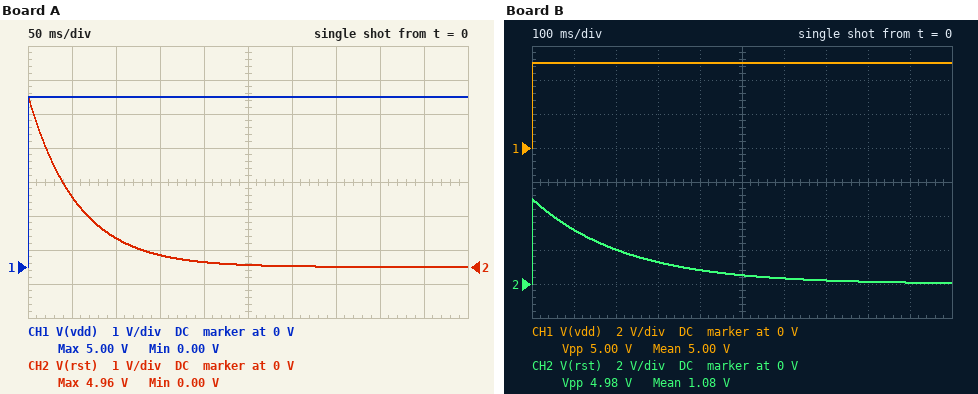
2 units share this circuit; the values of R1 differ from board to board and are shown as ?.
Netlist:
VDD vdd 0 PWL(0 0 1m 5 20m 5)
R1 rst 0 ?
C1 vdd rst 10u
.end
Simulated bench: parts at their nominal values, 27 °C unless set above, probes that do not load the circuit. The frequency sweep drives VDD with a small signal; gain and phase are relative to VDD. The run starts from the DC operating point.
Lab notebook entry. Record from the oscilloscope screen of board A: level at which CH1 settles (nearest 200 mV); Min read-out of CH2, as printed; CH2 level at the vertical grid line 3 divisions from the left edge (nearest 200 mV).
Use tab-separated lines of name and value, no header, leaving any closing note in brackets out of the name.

level at which CH1 settles	5.0 V
Min read-out of CH2, as printed	0.00 V
CH2 level at the vertical grid line 3 divisions from the left edge	400 mV
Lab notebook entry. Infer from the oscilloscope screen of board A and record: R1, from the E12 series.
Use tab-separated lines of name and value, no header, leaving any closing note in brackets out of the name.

R1, from the E12 series	5.6 kΩ
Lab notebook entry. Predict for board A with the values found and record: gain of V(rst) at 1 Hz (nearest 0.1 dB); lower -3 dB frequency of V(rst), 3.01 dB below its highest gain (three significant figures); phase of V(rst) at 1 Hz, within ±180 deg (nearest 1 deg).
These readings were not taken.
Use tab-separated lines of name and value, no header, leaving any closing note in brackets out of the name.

gain of V(rst) at 1 Hz	-9.6 dB
lower -3 dB frequency of V(rst), 3.01 dB below its highest gain	2.84 Hz
phase of V(rst) at 1 Hz, within ±180 deg	71 deg
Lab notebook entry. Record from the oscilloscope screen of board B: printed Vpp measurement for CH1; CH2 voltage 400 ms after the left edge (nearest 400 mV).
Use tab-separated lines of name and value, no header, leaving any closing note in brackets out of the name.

printed Vpp measurement for CH1	5.00 V
CH2 voltage 400 ms after the left edge	800 mV
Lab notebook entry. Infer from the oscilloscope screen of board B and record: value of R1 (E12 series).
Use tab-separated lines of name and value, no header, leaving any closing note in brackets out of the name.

value of R1	22 kΩ
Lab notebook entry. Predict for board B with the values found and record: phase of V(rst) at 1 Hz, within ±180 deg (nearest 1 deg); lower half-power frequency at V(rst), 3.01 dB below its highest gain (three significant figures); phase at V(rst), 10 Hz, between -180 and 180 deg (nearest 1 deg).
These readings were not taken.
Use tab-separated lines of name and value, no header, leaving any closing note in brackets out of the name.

phase of V(rst) at 1 Hz, within ±180 deg	36 deg
lower half-power frequency at V(rst), 3.01 dB below its highest gain	723 mHz
phase at V(rst), 10 Hz, between -180 and 180 deg	4 deg
